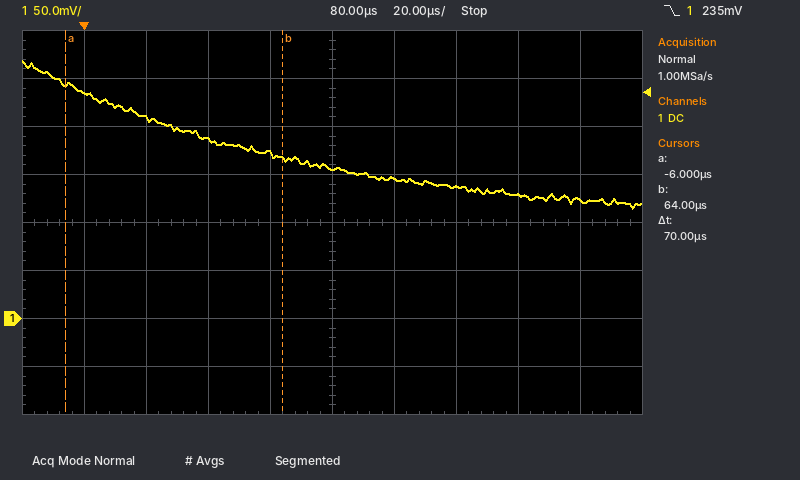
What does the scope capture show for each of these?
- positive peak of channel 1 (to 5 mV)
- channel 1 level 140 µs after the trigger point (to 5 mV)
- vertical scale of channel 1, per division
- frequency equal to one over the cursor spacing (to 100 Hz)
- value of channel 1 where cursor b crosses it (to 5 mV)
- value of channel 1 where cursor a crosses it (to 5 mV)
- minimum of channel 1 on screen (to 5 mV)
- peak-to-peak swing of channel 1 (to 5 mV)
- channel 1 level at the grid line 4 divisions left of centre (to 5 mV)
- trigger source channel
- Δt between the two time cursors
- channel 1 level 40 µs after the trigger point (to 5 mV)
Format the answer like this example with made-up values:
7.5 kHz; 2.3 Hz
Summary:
270 mV; 130 mV; 50 mV; 14.3 kHz; 165 mV; 245 mV; 115 mV; 155 mV; 235 mV; channel 1; 70 µs; 185 mV
